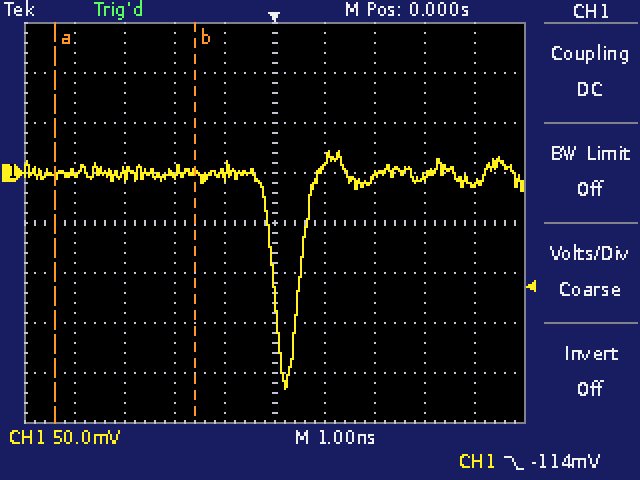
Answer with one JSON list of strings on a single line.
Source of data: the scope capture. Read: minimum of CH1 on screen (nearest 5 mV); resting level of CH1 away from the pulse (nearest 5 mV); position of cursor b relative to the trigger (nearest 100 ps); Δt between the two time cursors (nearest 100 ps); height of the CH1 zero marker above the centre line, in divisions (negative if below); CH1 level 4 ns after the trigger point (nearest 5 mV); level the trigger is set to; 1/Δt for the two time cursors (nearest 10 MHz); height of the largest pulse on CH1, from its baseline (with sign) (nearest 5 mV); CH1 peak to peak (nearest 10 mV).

["-215 mV", "0 mV", "-1.6 ns", "2.8 ns", "+1.0 div", "-10 mV", "-114 mV", "360 MHz", "-215 mV", "240 mV"]
